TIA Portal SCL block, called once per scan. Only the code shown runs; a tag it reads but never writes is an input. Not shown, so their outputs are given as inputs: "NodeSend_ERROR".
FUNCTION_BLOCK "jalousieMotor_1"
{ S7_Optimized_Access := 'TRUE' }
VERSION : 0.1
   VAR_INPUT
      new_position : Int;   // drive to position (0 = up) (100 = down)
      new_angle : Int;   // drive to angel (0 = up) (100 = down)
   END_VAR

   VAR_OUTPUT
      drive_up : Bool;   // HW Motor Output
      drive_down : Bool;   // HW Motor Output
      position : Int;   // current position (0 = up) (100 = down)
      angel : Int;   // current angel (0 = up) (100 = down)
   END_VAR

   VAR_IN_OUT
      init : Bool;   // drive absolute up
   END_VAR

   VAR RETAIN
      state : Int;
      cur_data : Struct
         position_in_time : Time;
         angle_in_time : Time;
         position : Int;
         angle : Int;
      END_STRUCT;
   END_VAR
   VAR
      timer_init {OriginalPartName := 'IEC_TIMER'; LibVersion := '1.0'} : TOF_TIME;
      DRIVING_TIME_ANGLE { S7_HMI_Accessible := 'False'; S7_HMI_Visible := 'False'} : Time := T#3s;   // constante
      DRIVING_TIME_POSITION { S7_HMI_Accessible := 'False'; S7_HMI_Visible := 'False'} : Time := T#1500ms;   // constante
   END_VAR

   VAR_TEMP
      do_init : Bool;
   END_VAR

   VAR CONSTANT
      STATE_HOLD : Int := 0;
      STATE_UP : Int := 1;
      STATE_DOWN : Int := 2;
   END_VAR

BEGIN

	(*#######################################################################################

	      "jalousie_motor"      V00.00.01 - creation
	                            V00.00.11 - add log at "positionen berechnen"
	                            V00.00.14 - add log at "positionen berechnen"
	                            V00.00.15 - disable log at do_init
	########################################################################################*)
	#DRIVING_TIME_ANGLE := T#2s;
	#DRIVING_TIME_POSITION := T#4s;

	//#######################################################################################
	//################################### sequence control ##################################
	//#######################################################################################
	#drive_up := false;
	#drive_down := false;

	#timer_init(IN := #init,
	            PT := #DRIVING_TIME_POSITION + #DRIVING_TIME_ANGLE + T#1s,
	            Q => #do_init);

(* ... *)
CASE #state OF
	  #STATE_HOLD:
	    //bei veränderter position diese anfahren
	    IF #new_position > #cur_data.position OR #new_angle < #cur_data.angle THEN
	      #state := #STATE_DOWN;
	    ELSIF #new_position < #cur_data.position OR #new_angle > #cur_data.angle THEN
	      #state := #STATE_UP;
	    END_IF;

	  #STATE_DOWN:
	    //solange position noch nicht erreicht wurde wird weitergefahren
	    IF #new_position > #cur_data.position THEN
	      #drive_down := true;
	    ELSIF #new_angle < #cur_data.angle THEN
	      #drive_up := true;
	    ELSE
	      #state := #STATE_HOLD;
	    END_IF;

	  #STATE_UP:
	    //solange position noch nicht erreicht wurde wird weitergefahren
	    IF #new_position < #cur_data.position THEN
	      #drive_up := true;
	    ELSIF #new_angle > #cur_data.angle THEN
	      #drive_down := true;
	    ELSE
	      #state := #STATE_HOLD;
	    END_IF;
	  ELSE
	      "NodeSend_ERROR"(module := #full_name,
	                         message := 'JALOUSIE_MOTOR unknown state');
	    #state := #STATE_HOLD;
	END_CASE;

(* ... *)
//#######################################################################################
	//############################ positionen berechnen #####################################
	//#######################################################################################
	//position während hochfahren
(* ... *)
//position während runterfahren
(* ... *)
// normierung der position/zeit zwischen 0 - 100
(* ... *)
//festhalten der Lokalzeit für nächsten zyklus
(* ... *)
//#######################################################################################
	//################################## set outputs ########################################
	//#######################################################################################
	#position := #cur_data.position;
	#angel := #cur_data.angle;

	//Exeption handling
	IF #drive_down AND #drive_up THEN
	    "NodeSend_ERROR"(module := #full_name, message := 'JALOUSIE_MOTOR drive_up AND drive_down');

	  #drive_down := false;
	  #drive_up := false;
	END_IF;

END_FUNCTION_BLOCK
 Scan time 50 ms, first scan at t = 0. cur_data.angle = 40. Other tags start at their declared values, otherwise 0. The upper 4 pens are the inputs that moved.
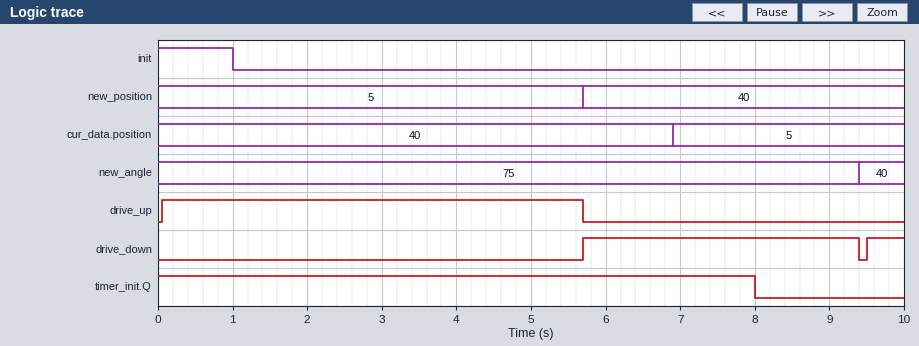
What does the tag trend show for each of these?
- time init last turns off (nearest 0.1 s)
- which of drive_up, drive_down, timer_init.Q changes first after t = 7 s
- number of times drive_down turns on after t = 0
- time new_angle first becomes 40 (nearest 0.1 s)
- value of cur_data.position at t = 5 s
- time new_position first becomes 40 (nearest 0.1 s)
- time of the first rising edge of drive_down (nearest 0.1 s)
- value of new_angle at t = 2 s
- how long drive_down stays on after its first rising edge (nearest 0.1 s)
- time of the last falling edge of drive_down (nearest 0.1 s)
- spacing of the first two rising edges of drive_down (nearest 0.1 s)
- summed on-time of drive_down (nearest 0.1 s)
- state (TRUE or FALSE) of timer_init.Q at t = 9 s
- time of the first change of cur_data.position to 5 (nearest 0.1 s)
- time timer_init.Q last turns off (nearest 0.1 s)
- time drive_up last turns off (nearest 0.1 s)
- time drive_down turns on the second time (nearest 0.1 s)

1.0 s
timer_init.Q
2
9.4 s
40
5.7 s
5.7 s
75
3.7 s
9.4 s
3.8 s
4.2 s
FALSE
6.9 s
8.0 s
5.7 s
9.5 s
